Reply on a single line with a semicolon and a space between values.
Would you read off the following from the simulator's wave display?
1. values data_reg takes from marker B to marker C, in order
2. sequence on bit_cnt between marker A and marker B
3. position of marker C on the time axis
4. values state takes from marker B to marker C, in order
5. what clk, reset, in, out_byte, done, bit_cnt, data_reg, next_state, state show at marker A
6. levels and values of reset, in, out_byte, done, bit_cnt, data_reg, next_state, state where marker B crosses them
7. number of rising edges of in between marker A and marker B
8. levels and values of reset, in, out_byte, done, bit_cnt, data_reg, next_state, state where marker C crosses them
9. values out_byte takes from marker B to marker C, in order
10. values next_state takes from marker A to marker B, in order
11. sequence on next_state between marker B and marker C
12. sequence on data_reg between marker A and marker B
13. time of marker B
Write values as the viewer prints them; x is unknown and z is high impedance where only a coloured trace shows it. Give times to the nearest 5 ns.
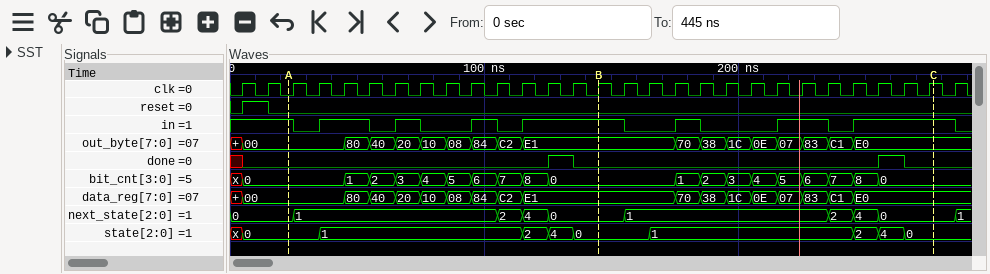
E1, 70, 38, 1C, 0E, 07, 83, C1, E0; 0, 1, 2, 3, 4, 5, 6, 7, 8, 0; 275 ns; 0, 1, 2, 4, 0; clk=0, reset=0, in=1, out_byte=00, done=0, bit_cnt=0, data_reg=00, next_state=0, state=0; reset=0, in=1, out_byte=E1, done=0, bit_cnt=0, data_reg=E1, next_state=0, state=0; 4; reset=0, in=1, out_byte=E0, done=0, bit_cnt=0, data_reg=E0, next_state=0, state=0; E1, 70, 38, 1C, 0E, 07, 83, C1, E0; 0, 1, 2, 4, 0; 0, 1, 2, 4, 0; 00, 80, 40, 20, 10, 08, 84, C2, E1; 145 ns
